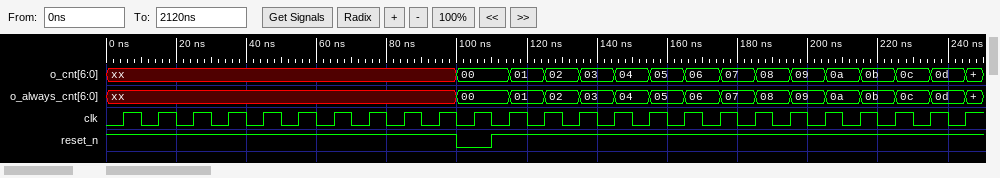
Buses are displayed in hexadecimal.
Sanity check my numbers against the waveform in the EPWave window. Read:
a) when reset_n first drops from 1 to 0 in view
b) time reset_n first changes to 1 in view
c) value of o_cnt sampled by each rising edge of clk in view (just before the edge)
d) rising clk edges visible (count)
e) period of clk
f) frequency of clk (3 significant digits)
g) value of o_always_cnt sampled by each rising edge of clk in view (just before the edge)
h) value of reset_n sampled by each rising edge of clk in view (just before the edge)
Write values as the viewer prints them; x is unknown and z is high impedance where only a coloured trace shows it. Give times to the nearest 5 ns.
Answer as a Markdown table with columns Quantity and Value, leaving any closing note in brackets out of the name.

| Quantity | Value |
|---|---|
| when reset_n first drops from 1 to 0 in view | 100 ns |
| time reset_n first changes to 1 in view | 110 ns |
| value of o_cnt sampled by each rising edge of clk in view | xx, xx, xx, xx, xx, xx, xx, xx, xx, xx, 00, 00, 01, 02, 03, 04, 05, 06, 07, 08, 09, 0a, 0b, 0c, 0d |
| rising clk edges visible | 25 |
| period of clk | 10 ns |
| frequency of clk | 100 MHz |
| value of o_always_cnt sampled by each rising edge of clk in view | xx, xx, xx, xx, xx, xx, xx, xx, xx, xx, 00, 00, 01, 02, 03, 04, 05, 06, 07, 08, 09, 0a, 0b, 0c, 0d |
| value of reset_n sampled by each rising edge of clk in view | 1 1 1 1 1 1 1 1 1 1 0 1 1 1 1 1 1 1 1 1 1 1 1 1 1 |
